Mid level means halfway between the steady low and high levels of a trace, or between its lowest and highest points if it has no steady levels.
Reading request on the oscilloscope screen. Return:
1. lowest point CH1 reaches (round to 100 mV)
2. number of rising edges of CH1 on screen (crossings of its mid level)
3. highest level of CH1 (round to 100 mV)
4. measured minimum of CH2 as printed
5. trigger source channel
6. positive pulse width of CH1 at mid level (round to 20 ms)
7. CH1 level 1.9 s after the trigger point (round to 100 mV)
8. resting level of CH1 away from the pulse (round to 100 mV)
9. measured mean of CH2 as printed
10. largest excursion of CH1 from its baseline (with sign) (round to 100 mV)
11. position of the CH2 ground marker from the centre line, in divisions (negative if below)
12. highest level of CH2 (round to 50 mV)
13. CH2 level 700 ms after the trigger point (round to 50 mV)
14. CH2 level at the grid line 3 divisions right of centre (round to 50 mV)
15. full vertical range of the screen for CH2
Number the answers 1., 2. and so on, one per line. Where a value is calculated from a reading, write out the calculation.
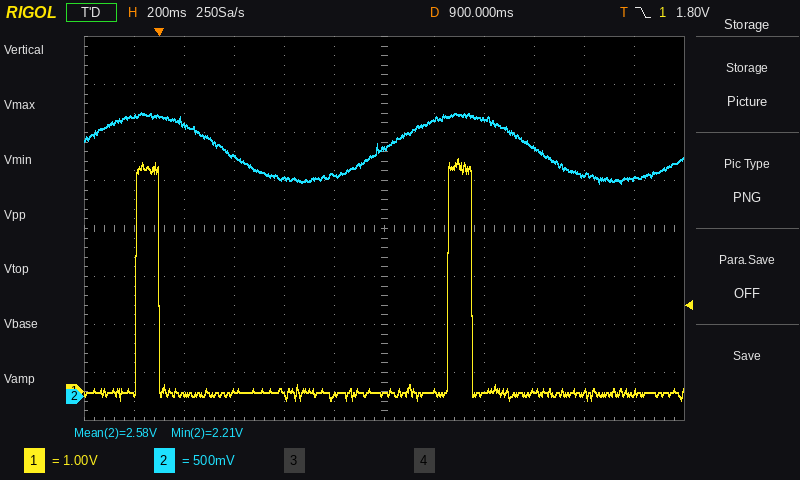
1. -200 mV
2. 2
3. 4.9 V
4. 2.21 V
5. CH1
6. 100 ms
7. 0.0 V
8. 0.0 V
9. 2.58 V
10. 4.9 V − (0.0 V) = +4.9 V
11. -3.5 div
12. 2.95 V
13. 2.30 V
14. 2.60 V
15. 4 V
